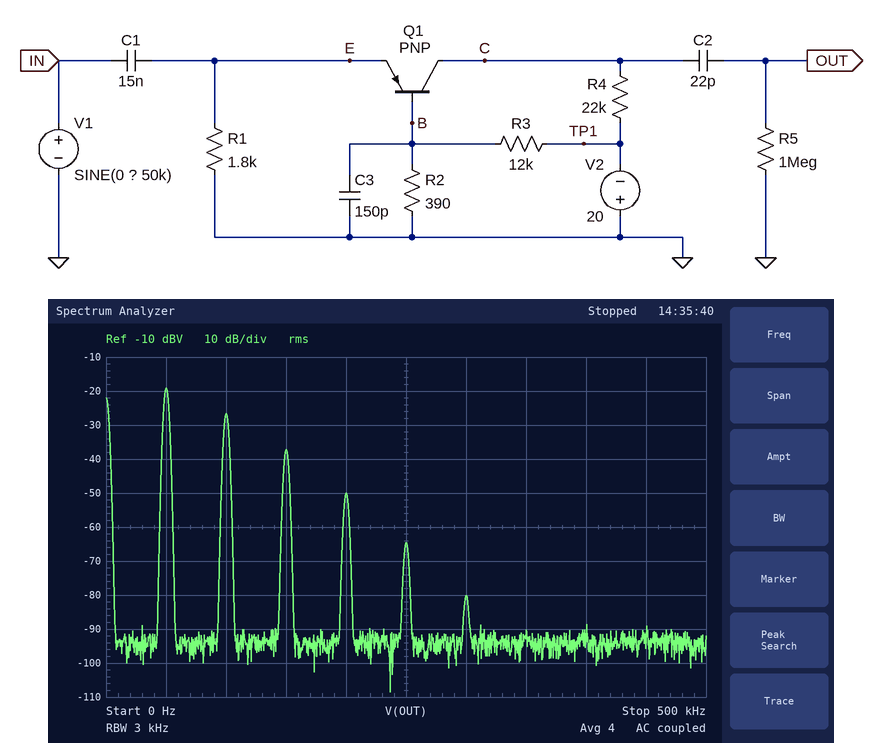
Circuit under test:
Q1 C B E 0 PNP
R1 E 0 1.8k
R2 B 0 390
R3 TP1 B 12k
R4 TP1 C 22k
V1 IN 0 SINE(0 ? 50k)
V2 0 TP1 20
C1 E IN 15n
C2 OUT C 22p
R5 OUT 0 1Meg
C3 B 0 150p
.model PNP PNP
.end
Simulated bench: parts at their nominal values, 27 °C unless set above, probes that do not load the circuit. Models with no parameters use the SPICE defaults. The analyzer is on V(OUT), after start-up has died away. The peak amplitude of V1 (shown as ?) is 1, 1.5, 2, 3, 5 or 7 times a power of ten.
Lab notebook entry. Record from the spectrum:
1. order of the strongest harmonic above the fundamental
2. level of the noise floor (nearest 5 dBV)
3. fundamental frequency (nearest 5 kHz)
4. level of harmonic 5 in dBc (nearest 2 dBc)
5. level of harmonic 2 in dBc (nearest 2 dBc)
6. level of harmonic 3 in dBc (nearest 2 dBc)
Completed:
2
-95 dBV
50 kHz
-46 dBc
-8 dBc
-18 dBc
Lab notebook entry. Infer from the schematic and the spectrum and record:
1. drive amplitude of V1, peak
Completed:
50 mV
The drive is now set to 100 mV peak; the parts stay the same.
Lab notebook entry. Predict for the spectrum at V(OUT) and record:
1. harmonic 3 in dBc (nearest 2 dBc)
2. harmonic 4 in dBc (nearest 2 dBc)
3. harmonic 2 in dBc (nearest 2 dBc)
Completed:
-10 dBc
-18 dBc
-4 dBc
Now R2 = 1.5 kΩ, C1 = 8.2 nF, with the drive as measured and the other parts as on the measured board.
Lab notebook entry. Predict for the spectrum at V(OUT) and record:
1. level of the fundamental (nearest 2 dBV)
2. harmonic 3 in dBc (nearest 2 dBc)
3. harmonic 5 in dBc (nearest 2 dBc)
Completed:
2 dBV
-20 dBc
-26 dBc
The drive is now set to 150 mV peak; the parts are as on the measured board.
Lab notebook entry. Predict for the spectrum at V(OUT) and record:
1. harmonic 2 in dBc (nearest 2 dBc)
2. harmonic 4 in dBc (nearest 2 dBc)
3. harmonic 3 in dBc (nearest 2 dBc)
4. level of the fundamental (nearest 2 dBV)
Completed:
-2 dBc
-12 dBc
-6 dBc
-2 dBV
